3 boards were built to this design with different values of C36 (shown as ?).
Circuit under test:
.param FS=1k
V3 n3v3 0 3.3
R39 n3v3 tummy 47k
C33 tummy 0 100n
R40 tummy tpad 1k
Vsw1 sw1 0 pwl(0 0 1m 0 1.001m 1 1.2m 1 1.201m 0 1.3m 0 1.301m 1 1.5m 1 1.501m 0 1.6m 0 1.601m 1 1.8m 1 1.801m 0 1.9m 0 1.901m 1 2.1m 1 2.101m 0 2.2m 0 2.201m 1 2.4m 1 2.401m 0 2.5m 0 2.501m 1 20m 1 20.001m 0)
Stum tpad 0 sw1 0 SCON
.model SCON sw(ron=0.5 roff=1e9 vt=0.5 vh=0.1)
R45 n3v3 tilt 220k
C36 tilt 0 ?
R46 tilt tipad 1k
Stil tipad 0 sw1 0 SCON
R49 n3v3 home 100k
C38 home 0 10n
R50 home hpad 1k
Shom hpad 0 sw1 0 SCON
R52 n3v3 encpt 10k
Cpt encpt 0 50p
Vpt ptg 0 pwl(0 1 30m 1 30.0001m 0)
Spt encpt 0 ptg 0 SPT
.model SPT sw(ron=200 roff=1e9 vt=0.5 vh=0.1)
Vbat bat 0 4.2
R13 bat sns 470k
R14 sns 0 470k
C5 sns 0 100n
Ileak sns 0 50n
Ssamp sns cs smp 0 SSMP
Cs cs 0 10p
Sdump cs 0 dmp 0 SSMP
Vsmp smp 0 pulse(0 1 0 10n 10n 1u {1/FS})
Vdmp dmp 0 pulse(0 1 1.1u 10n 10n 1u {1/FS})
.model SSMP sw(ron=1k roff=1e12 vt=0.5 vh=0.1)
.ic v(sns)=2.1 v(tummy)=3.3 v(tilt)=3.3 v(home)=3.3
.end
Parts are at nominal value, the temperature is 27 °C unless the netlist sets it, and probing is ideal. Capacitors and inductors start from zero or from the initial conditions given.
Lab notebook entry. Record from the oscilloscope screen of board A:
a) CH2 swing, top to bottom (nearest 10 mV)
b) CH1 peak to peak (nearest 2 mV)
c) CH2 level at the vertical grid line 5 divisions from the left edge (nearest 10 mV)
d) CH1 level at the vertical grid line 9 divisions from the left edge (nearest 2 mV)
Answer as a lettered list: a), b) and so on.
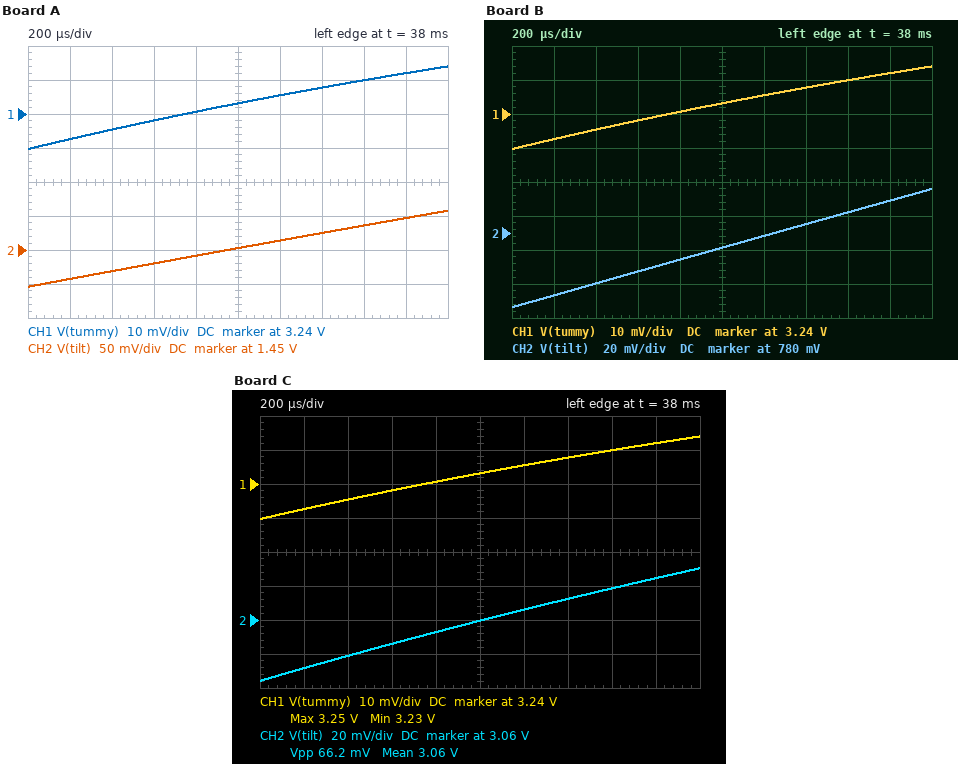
a) 110 mV
b) 24 mV
c) 1.45 V
d) 3.252 V
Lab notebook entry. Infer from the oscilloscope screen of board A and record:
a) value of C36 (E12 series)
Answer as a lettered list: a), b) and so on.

a) 150 nF
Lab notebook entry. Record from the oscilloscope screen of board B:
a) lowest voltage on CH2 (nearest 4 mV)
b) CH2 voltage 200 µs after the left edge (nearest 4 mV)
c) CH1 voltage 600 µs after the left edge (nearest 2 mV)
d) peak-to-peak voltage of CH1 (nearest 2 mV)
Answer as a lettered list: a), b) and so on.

a) 736 mV
b) 744 mV
c) 3.238 V
d) 24 mV
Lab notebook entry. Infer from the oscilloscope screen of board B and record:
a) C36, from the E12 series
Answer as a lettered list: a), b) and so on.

a) 330 nF
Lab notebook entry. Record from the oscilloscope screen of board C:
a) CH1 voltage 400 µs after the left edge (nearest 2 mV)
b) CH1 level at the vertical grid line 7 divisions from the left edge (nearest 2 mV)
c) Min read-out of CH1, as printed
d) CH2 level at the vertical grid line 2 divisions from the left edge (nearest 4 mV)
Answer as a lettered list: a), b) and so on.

a) 3.236 V
b) 3.248 V
c) 3.23 V
d) 3.040 V
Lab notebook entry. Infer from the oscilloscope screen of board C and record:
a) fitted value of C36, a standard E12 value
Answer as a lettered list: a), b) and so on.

a) 33 nF
